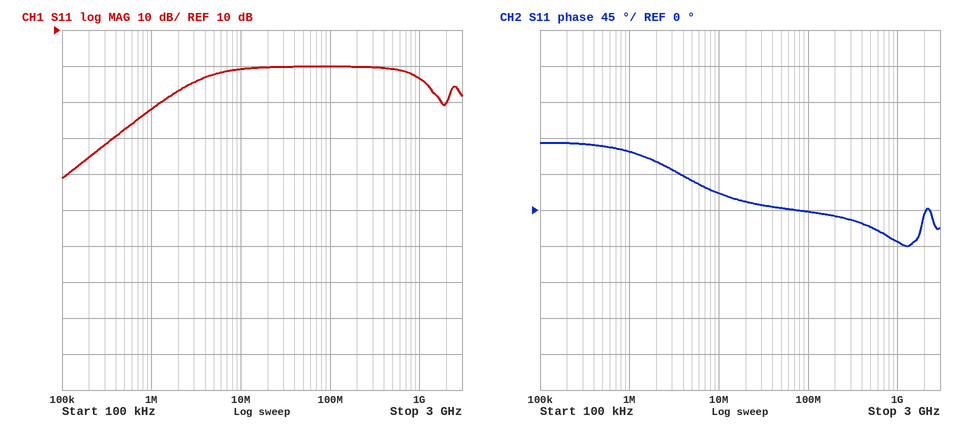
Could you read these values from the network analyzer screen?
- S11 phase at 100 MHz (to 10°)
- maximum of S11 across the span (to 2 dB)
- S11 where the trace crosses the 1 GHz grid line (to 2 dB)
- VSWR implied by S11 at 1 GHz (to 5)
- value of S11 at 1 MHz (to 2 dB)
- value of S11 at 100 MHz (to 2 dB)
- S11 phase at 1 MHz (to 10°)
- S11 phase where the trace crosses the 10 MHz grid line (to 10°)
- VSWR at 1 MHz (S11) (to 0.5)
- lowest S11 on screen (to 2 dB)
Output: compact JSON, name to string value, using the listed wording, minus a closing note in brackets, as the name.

{"S11 phase at 100 MHz": "0°", "maximum of S11 across the span": "0 dB", "S11 where the trace crosses the 1 GHz grid line": "-4 dB", "VSWR implied by S11 at 1 GHz": "5", "value of S11 at 1 MHz": "-12 dB", "value of S11 at 100 MHz": "0 dB", "S11 phase at 1 MHz": "70°", "S11 phase where the trace crosses the 10 MHz grid line": "20°", "VSWR at 1 MHz (S11)": "1.5", "lowest S11 on screen": "-32 dB"}
